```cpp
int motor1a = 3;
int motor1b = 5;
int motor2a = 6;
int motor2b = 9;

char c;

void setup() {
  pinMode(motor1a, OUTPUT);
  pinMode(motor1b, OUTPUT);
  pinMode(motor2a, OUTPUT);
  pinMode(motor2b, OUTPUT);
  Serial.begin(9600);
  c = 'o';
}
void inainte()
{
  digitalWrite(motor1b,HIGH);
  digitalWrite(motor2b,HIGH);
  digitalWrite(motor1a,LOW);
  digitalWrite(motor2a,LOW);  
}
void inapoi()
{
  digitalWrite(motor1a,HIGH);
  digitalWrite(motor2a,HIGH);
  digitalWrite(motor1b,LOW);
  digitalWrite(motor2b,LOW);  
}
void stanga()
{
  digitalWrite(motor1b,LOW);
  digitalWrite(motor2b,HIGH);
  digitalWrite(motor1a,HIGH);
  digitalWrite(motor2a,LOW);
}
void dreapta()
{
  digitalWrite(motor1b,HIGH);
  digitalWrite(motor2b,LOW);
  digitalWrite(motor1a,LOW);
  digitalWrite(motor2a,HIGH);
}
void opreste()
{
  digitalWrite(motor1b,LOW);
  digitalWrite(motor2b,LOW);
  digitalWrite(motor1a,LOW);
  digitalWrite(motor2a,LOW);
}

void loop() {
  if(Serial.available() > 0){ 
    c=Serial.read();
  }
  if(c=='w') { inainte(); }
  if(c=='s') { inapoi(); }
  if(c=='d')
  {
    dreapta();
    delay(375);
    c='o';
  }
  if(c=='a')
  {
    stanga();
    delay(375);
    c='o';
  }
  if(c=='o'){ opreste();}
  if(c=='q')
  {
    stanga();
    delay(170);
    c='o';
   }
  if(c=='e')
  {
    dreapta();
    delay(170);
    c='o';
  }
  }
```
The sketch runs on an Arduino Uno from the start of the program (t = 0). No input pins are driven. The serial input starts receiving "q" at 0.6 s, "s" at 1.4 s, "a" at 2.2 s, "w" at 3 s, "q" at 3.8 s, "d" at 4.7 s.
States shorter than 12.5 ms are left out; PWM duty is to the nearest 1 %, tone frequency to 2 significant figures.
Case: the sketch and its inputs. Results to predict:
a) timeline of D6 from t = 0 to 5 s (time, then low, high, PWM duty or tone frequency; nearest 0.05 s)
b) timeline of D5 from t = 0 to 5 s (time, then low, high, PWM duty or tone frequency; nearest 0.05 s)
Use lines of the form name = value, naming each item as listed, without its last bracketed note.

timeline of D6 from t = 0 to 5 s = 0 s low; 1.4 s high; 2.2 s low; 4.7 s high
timeline of D5 from t = 0 to 5 s = 0 s low; 3 s high; 3.8 s low; 4.7 s high
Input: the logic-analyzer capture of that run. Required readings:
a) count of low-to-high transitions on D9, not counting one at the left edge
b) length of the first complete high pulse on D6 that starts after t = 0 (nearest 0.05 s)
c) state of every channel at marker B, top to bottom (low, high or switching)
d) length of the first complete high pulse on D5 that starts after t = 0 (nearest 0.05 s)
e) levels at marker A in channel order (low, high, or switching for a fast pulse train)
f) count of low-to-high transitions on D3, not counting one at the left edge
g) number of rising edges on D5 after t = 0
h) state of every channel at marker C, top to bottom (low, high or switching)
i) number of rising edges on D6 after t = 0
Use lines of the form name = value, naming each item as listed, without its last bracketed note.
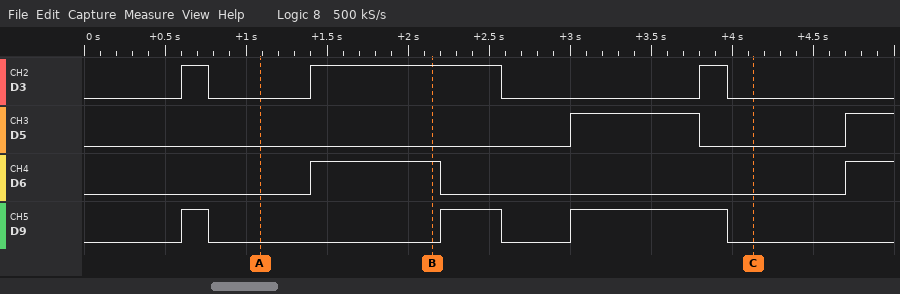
count of low-to-high transitions on D9, not counting one at the left edge = 3
length of the first complete high pulse on D6 that starts after t = 0 = 0.80 s
state of every channel at marker B, top to bottom = D3 high, D5 low, D6 high, D9 low
length of the first complete high pulse on D5 that starts after t = 0 = 0.80 s
levels at marker A in channel order = D3 low, D5 low, D6 low, D9 low
count of low-to-high transitions on D3, not counting one at the left edge = 3
number of rising edges on D5 after t = 0 = 2
state of every channel at marker C, top to bottom = D3 low, D5 low, D6 low, D9 low
number of rising edges on D6 after t = 0 = 2
